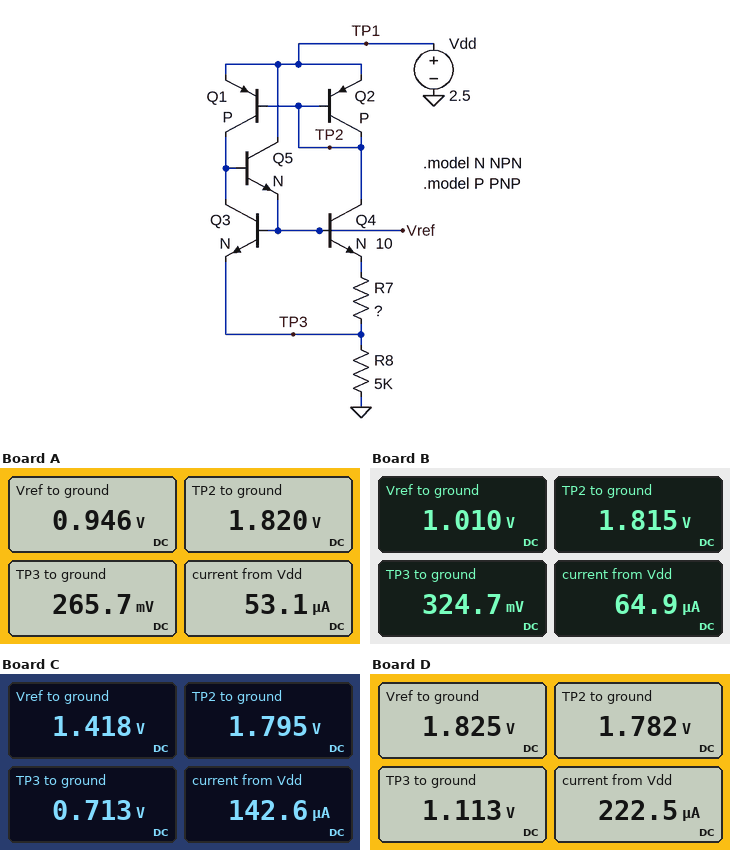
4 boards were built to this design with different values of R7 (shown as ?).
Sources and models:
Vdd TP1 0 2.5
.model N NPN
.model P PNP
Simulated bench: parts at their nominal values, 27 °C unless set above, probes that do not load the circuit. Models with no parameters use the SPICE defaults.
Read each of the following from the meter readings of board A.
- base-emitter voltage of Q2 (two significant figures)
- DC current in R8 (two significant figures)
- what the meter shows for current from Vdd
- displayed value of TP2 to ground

-680 mV
53 µA
53.1 µA
1.820 V
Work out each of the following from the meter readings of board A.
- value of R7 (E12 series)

2.2 kΩ
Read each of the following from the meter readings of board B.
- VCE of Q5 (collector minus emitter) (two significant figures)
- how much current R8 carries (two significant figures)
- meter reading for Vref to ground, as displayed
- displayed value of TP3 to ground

1.5 V
65 µA
1.010 V
324.7 mV
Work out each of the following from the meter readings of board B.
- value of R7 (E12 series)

1.8 kΩ
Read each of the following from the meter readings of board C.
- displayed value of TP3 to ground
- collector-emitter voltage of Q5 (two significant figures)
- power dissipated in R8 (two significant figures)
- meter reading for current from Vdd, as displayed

0.713 V
1.1 V
100 µW
142.6 µA
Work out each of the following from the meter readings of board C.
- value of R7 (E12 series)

820 Ω
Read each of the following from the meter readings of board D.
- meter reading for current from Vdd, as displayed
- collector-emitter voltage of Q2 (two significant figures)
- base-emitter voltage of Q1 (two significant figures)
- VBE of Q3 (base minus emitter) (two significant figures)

222.5 µA
-720 mV
-720 mV
710 mV
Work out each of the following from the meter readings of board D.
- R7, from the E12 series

390 Ω
